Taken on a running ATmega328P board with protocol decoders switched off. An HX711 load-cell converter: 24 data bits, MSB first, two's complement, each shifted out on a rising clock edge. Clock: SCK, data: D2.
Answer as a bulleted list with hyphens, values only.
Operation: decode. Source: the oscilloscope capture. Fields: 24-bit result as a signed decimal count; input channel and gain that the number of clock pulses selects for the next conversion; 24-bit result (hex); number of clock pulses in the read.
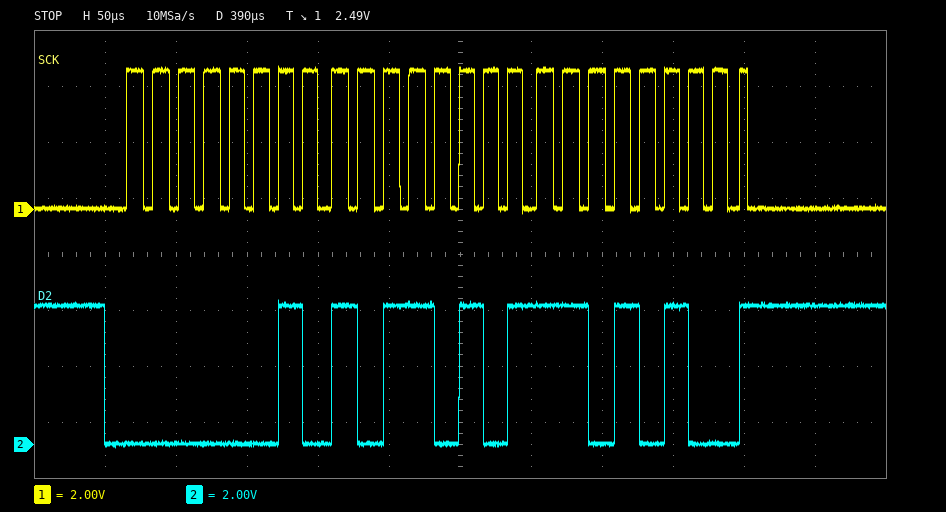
- 177620
- channel A, gain 128
- 0x02B5D4
- 25
